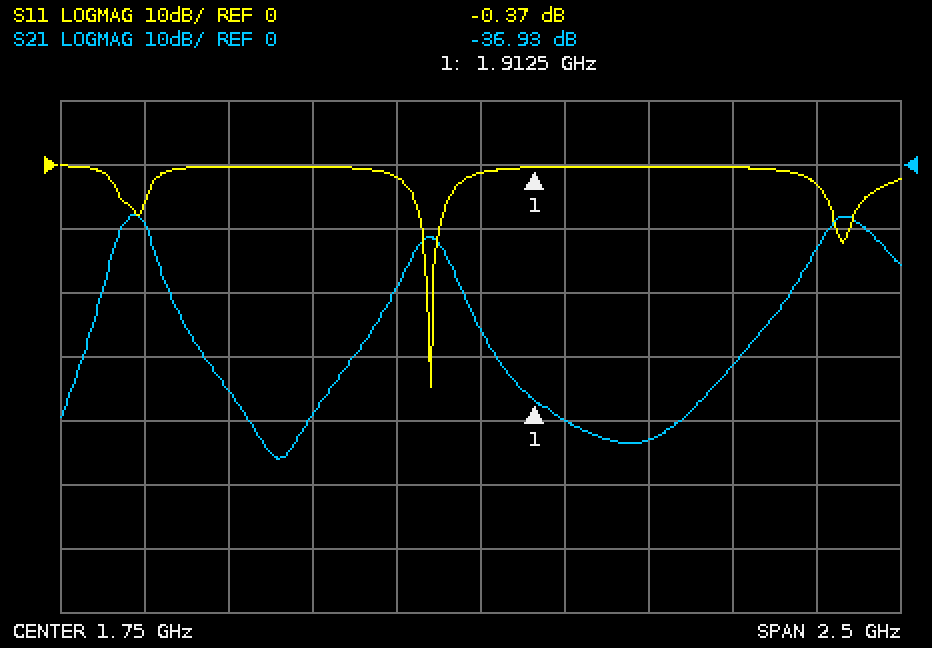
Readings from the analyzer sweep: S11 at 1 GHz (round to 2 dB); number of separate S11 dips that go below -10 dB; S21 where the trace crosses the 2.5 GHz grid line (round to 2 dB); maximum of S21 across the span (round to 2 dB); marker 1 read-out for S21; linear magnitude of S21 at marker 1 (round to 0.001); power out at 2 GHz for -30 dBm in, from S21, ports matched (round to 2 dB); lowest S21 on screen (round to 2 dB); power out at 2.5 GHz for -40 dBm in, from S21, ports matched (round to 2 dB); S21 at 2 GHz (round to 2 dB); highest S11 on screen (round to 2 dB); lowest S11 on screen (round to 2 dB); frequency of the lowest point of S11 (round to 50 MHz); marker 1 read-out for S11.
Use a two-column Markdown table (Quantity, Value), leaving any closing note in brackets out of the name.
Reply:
| Quantity | Value |
|---|---|
| S11 at 1 GHz | 0 dB |
| number of separate S11 dips that go below -10 dB | 2 |
| S21 where the trace crosses the 2.5 GHz grid line | -32 dB |
| maximum of S21 across the span | -8 dB |
| marker 1 read-out for S21 | -36.93 dB |
| linear magnitude of S21 at marker 1 | 0.014 |
| power out at 2 GHz for -30 dBm in, from S21, ports matched | -70 dBm |
| lowest S21 on screen | -46 dB |
| power out at 2.5 GHz for -40 dBm in, from S21, ports matched | -72 dBm |
| S21 at 2 GHz | -40 dB |
| highest S11 on screen | 0 dB |
| lowest S11 on screen | -34 dB |
| frequency of the lowest point of S11 | 1.60 GHz |
| marker 1 read-out for S11 | -0.37 dB |
